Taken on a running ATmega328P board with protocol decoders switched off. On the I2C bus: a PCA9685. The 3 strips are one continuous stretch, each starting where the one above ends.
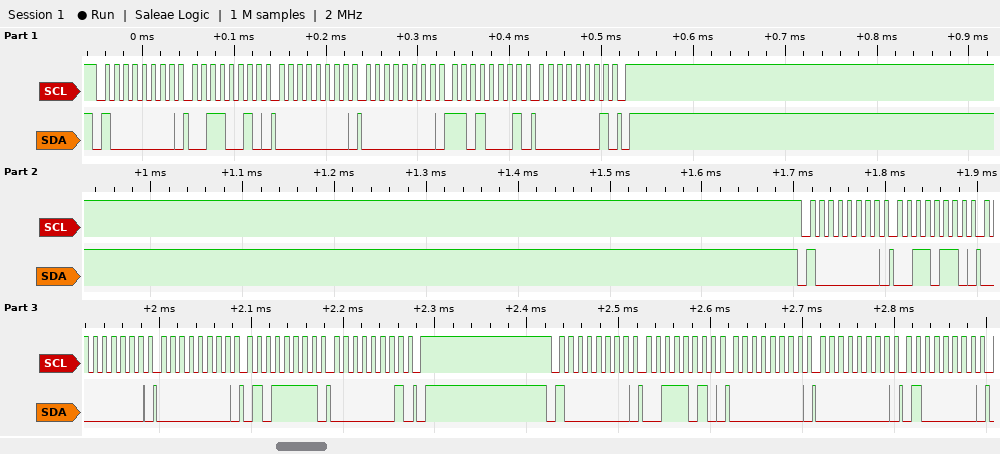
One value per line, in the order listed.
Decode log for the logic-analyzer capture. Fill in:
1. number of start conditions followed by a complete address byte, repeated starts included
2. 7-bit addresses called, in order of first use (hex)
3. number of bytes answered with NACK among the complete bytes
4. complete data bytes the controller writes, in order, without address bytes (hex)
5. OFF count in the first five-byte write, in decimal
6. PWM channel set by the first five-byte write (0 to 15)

3
0x40
0
32 00 00 D1 01 36 00 00 5F 01 3A 00 00 40
465
11
